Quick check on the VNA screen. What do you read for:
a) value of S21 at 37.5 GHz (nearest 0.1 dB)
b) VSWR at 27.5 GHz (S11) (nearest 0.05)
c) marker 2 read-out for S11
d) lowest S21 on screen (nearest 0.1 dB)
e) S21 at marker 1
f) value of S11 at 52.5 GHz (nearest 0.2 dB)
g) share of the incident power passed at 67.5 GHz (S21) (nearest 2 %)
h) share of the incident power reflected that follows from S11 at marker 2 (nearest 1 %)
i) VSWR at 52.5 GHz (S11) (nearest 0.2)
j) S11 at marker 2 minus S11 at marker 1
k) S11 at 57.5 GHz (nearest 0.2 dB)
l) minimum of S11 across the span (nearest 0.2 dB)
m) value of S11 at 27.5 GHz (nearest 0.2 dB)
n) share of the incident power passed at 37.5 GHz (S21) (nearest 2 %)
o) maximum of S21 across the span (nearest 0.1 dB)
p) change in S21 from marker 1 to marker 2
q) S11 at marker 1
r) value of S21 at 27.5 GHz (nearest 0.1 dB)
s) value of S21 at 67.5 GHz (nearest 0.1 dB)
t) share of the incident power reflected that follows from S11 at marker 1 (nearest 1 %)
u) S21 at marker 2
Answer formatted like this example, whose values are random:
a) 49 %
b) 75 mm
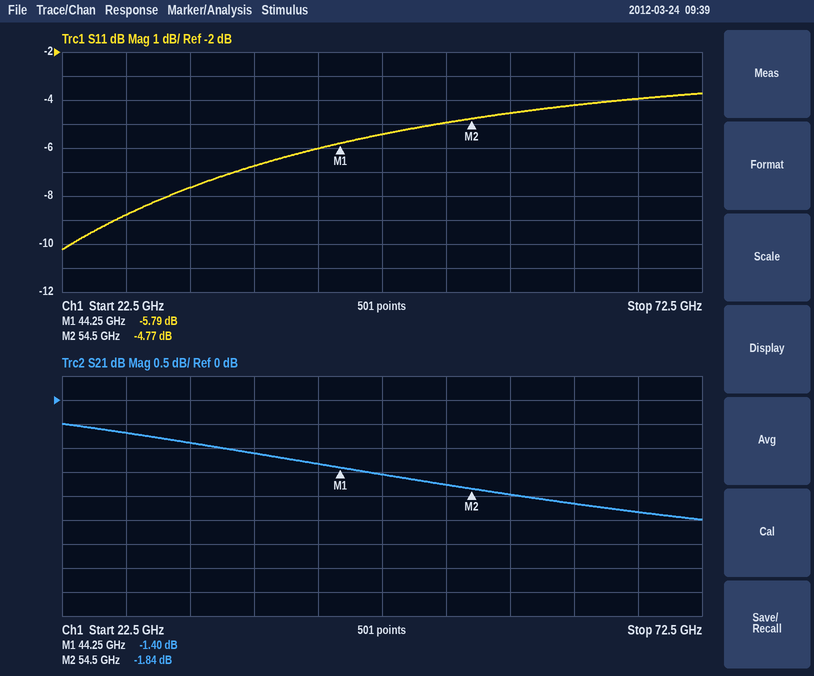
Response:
a) -1.1 dB
b) 2.15
c) -4.77 dB
d) -2.5 dB
e) -1.40 dB
f) -5.0 dB
g) 58 %
h) 33 %
i) 3.6
j) 1.02 dB
k) -4.6 dB
l) -10.2 dB
m) -8.8 dB
n) 78 %
o) -0.5 dB
p) -0.44 dB
q) -5.79 dB
r) -0.7 dB
s) -2.3 dB
t) 26 %
u) -1.84 dB
